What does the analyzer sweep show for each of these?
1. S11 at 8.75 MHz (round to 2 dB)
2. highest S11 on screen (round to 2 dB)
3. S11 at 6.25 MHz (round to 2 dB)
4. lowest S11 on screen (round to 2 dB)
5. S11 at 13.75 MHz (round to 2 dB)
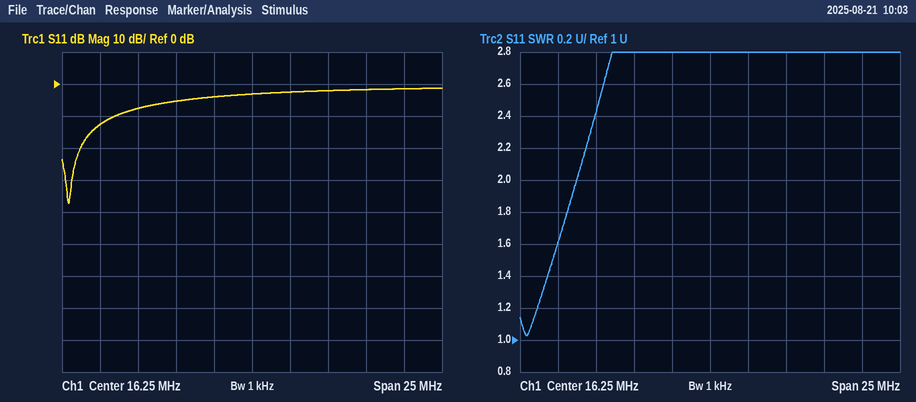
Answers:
-8 dB
-2 dB
-12 dB
-38 dB
-4 dB
